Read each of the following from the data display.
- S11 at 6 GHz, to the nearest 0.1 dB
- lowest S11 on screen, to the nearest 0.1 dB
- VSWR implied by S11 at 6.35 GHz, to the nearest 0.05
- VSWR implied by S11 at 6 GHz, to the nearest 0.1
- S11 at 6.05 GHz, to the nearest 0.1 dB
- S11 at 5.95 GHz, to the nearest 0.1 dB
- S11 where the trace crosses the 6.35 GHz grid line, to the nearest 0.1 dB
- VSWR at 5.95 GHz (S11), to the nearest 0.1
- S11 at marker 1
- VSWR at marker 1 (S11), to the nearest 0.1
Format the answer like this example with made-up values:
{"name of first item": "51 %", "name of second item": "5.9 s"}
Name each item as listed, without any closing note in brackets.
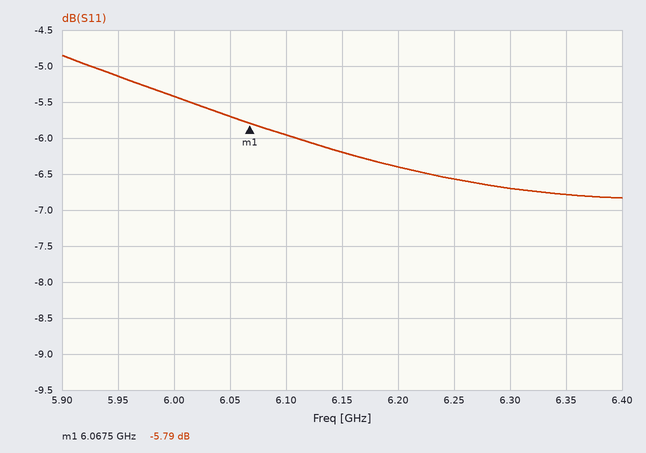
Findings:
{"S11 at 6 GHz, to the nearest 0.1 dB": "-5.4 dB", "lowest S11 on screen, to the nearest 0.1 dB": "-6.8 dB", "VSWR implied by S11 at 6.35 GHz, to the nearest 0.05": "2.70", "VSWR implied by S11 at 6 GHz, to the nearest 0.1": "3.3", "S11 at 6.05 GHz, to the nearest 0.1 dB": "-5.7 dB", "S11 at 5.95 GHz, to the nearest 0.1 dB": "-5.1 dB", "S11 where the trace crosses the 6.35 GHz grid line, to the nearest 0.1 dB": "-6.8 dB", "VSWR at 5.95 GHz (S11), to the nearest 0.1": "3.5", "S11 at marker 1": "-5.79 dB", "VSWR at marker 1 (S11), to the nearest 0.1": "3.1"}
